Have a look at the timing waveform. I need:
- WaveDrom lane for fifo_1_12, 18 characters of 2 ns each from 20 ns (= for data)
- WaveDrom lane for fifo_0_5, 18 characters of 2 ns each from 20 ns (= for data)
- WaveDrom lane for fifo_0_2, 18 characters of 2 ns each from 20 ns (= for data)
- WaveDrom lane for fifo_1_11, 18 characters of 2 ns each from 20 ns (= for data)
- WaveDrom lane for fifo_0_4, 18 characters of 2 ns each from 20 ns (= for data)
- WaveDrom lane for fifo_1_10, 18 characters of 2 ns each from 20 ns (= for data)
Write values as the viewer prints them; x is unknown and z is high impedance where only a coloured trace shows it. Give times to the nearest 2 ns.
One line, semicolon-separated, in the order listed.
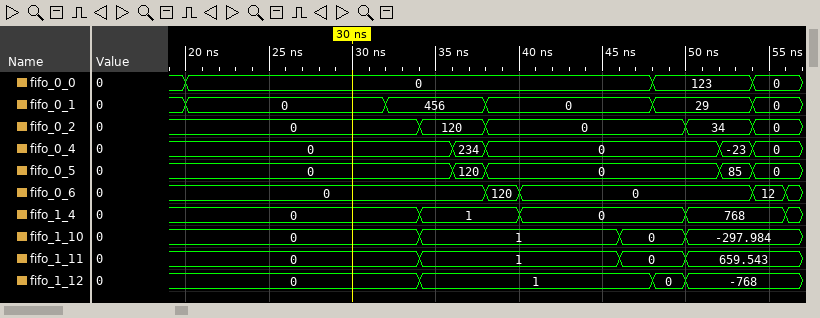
{name: 'fifo_1_12', wave: '=......=......==..', data: '0 1 0 -768'}; {name: 'fifo_0_5', wave: '=.......==......==', data: '0 120 0 85 0'}; {name: 'fifo_0_2', wave: '=......=.=.....=.=', data: '0 120 0 34 0'}; {name: 'fifo_1_11', wave: '=......=.....=.=..', data: '0 1 0 659.543'}; {name: 'fifo_0_4', wave: '=.......==......==', data: '0 234 0 -23 0'}; {name: 'fifo_1_10', wave: '=......=.....=.=..', data: '0 1 0 -297.984'}
